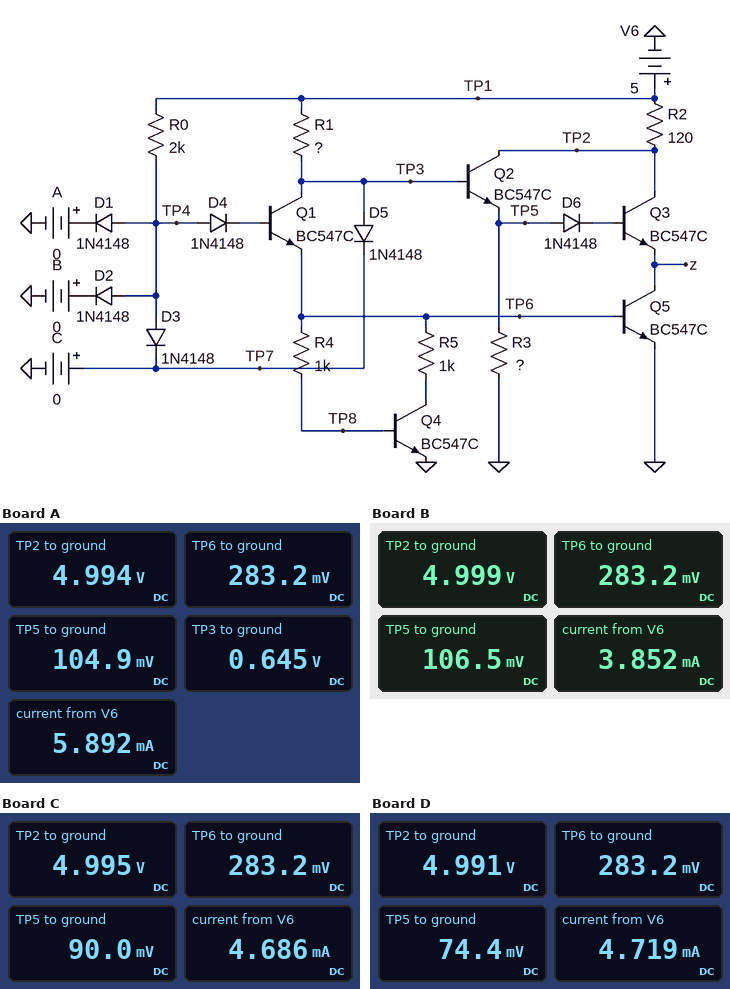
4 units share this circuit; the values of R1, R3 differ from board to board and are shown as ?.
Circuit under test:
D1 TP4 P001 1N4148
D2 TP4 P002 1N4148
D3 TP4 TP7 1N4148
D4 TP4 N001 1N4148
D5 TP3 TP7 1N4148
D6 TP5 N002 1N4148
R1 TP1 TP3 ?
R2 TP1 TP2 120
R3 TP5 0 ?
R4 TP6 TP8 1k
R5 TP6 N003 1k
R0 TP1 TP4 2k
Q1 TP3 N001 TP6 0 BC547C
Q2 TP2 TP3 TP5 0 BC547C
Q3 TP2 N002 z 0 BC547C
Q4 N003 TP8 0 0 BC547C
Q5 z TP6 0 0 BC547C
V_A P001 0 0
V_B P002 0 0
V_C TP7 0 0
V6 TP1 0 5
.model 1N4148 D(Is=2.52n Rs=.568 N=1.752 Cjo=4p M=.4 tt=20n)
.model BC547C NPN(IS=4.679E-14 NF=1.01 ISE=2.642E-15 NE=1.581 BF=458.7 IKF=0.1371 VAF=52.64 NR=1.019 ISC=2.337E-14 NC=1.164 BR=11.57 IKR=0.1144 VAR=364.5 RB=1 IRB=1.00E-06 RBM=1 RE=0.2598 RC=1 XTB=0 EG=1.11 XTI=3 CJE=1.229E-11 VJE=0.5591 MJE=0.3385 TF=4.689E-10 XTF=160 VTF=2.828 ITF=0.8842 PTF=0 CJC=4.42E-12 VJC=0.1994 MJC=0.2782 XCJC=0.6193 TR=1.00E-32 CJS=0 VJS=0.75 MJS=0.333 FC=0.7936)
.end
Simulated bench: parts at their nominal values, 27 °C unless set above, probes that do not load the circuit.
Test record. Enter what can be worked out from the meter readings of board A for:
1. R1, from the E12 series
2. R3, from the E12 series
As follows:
1.2 kΩ
2.2 kΩ
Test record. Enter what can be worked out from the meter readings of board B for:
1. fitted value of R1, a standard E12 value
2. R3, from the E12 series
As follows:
2.7 kΩ
10 kΩ
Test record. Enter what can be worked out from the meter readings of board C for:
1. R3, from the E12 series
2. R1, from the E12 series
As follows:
2.2 kΩ
1.8 kΩ
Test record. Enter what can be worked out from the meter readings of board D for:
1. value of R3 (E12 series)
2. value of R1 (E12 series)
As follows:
1 kΩ
1.8 kΩ
